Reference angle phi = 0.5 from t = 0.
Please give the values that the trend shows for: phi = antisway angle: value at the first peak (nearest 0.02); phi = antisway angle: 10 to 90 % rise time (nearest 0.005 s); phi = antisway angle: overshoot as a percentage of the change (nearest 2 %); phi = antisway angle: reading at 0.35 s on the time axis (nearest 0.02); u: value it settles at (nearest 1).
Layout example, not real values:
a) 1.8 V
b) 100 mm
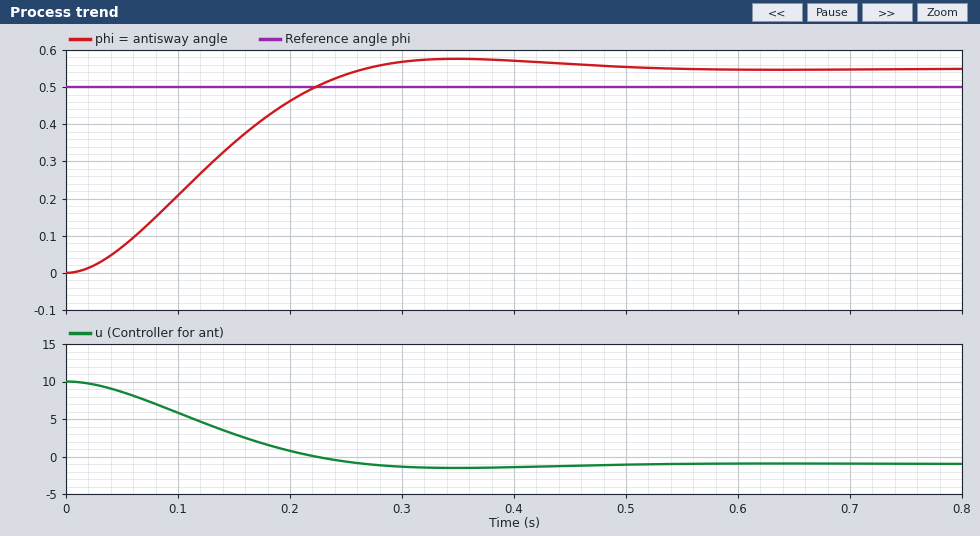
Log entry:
a) 0.58
b) 0.175 s
c) 4 %
d) 0.58
e) -1
